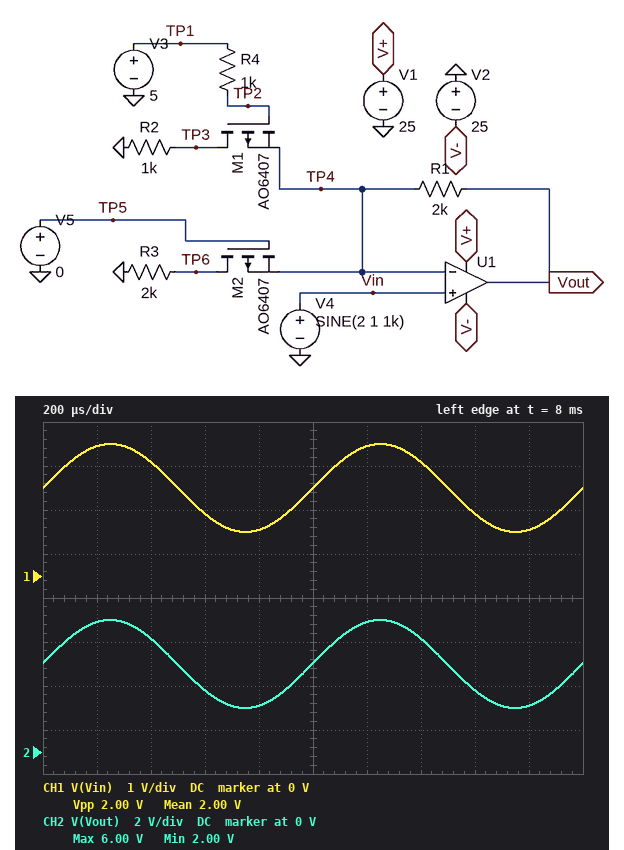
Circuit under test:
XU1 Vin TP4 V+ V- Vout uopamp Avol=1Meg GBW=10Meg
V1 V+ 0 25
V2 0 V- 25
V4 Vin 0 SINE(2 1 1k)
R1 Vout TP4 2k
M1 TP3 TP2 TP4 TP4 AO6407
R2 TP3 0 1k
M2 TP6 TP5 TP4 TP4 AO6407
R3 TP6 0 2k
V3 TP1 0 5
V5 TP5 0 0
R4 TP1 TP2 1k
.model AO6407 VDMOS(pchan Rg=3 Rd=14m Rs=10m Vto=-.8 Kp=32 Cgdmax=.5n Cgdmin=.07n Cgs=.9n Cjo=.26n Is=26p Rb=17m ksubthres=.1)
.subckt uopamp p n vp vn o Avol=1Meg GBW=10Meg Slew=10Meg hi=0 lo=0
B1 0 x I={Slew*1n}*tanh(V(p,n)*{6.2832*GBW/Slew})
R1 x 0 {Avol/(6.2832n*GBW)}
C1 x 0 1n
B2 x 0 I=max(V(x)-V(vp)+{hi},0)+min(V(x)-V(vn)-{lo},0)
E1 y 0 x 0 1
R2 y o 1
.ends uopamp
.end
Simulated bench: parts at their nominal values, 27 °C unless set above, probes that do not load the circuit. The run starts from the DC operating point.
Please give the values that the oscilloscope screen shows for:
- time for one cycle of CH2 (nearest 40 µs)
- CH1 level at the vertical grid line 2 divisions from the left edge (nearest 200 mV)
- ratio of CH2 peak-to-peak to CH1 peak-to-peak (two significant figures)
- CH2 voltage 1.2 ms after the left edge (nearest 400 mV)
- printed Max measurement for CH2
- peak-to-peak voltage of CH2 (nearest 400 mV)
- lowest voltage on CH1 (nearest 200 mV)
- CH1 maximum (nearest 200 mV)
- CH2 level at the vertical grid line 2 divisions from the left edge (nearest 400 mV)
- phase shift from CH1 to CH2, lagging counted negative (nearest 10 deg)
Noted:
1.00 ms
2.6 V
2.0
6.0 V
6.00 V
4.0 V
1.0 V
3.0 V
5.2 V
0 deg
